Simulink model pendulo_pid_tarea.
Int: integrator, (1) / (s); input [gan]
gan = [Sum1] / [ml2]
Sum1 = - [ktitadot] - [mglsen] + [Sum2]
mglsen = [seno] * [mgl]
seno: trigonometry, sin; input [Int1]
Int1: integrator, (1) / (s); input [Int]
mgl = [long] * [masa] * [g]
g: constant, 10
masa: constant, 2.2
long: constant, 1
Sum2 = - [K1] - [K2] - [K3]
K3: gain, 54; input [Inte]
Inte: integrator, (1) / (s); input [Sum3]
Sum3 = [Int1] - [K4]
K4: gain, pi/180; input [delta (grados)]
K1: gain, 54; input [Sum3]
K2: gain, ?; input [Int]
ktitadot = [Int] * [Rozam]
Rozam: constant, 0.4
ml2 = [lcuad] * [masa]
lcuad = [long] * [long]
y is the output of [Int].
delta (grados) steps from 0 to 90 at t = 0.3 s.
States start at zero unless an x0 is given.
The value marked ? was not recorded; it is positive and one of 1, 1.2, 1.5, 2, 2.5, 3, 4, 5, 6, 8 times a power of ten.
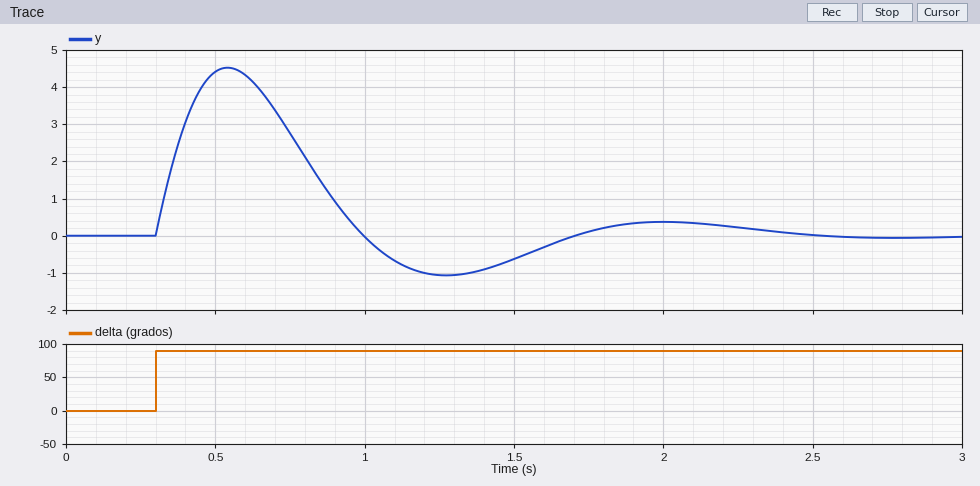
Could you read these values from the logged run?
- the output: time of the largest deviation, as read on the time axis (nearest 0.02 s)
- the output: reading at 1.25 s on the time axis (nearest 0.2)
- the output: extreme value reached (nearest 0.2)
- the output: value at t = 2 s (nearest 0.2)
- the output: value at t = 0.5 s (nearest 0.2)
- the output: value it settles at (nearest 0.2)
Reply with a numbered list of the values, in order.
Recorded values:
1. 0.54 s
2. -1.0
3. 4.6
4. 0.4
5. 4.4
6. 0.0
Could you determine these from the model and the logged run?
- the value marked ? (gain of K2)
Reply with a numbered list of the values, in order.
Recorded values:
1. 10
